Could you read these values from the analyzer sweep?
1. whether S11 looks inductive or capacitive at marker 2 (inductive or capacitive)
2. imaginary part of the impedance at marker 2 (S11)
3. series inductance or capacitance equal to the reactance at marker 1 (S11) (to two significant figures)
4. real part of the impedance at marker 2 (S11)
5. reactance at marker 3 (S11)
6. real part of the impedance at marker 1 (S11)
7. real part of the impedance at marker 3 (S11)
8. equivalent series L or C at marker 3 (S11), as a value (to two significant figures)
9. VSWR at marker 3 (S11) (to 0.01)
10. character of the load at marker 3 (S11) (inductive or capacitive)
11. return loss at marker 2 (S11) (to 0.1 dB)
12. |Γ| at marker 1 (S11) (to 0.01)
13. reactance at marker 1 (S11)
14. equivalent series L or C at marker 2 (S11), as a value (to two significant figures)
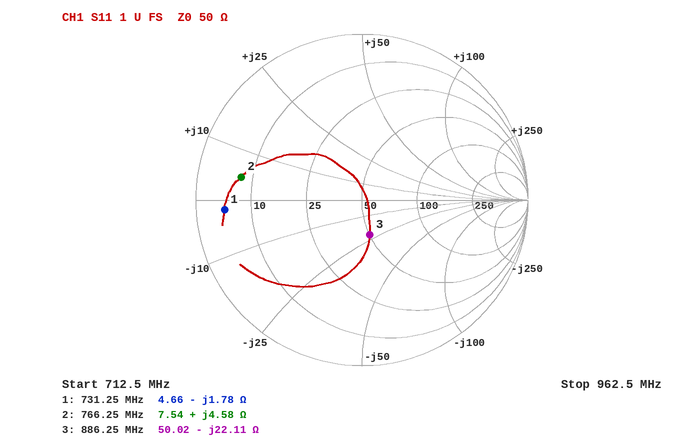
inductive
+4.58 Ω
120 pF
7.54 Ω
-22.11 Ω
4.66 Ω
50.02 Ω
8.1 pF
1.55
capacitive
2.6 dB
0.83
-1.78 Ω
950 pH
